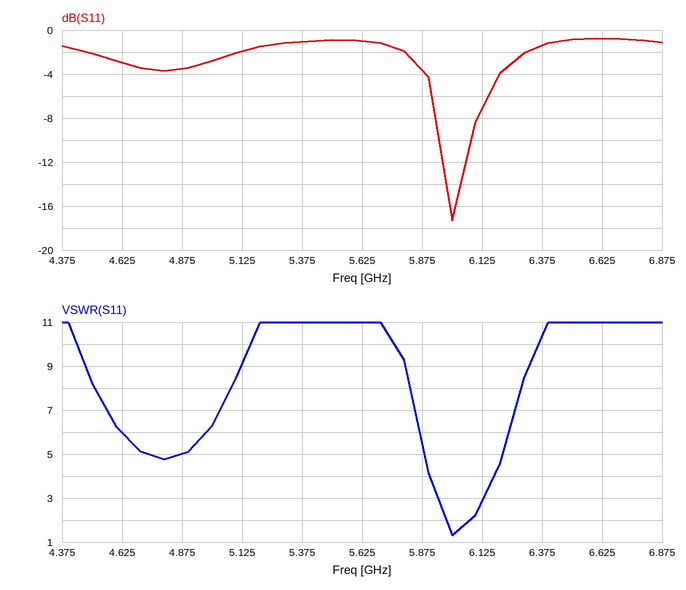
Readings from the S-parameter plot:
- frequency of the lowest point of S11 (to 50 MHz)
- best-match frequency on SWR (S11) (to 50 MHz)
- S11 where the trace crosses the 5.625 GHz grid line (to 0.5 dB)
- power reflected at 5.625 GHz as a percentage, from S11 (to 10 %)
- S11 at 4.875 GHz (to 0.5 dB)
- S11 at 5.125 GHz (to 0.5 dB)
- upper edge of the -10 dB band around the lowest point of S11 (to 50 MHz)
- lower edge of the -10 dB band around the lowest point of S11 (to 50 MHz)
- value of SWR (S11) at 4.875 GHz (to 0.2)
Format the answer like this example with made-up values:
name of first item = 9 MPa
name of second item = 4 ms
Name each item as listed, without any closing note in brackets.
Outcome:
frequency of the lowest point of S11 = 6.00 GHz
best-match frequency on SWR (S11) = 6.00 GHz
S11 where the trace crosses the 5.625 GHz grid line = -1.0 dB
power reflected at 5.625 GHz as a percentage, from S11 = 80 %
S11 at 4.875 GHz = -3.5 dB
S11 at 5.125 GHz = -2.0 dB
upper edge of the -10 dB band around the lowest point of S11 = 6.10 GHz
lower edge of the -10 dB band around the lowest point of S11 = 5.95 GHz
value of SWR (S11) at 4.875 GHz = 5.0
